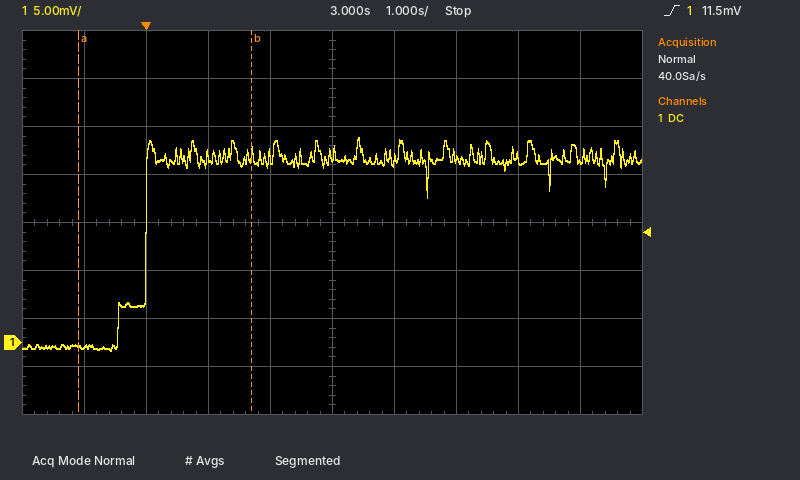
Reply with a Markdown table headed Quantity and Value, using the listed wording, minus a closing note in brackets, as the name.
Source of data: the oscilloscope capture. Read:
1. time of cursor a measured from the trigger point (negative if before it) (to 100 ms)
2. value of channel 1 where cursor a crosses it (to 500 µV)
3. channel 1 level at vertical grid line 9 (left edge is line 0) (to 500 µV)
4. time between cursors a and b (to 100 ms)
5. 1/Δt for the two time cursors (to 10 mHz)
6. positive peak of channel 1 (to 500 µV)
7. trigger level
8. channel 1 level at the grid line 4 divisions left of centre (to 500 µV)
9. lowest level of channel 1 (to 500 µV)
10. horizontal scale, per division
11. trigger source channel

| Quantity | Value |
|---|---|
| time of cursor a measured from the trigger point (negative if before it) | -1.1 s |
| value of channel 1 where cursor a crosses it | -500 µV |
| channel 1 level at vertical grid line 9 (left edge is line 0) | 19.0 mV |
| time between cursors a and b | 2.8 s |
| 1/Δt for the two time cursors | 360 mHz |
| positive peak of channel 1 | 21.5 mV |
| trigger level | 11.5 mV |
| channel 1 level at the grid line 4 divisions left of centre | -500 µV |
| lowest level of channel 1 | -1.0 mV |
| horizontal scale, per division | 1 s |
| trigger source channel | channel 1 |
